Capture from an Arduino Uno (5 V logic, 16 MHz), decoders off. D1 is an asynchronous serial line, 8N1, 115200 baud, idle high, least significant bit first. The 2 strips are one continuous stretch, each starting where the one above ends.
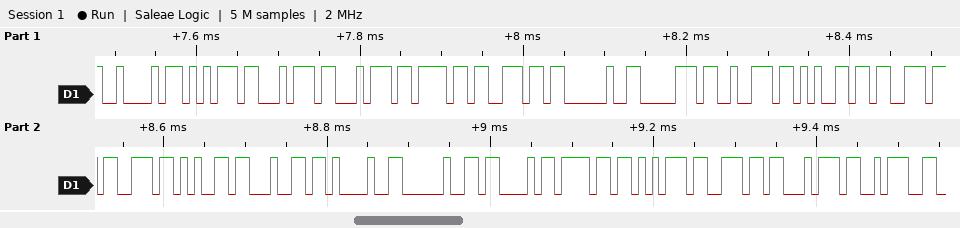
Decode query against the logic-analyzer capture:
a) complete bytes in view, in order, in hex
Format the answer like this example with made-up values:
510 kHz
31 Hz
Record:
42 75 74 74 6F 6E 20 70 72 65 73 73 65 64 21 20 43 6F 75 6E 74 3A
